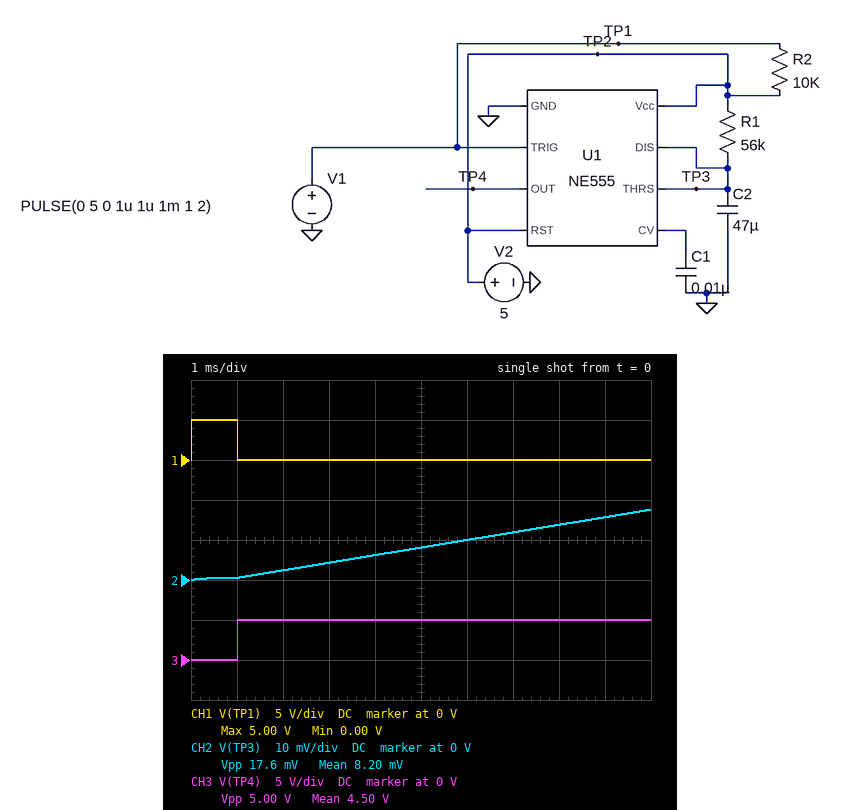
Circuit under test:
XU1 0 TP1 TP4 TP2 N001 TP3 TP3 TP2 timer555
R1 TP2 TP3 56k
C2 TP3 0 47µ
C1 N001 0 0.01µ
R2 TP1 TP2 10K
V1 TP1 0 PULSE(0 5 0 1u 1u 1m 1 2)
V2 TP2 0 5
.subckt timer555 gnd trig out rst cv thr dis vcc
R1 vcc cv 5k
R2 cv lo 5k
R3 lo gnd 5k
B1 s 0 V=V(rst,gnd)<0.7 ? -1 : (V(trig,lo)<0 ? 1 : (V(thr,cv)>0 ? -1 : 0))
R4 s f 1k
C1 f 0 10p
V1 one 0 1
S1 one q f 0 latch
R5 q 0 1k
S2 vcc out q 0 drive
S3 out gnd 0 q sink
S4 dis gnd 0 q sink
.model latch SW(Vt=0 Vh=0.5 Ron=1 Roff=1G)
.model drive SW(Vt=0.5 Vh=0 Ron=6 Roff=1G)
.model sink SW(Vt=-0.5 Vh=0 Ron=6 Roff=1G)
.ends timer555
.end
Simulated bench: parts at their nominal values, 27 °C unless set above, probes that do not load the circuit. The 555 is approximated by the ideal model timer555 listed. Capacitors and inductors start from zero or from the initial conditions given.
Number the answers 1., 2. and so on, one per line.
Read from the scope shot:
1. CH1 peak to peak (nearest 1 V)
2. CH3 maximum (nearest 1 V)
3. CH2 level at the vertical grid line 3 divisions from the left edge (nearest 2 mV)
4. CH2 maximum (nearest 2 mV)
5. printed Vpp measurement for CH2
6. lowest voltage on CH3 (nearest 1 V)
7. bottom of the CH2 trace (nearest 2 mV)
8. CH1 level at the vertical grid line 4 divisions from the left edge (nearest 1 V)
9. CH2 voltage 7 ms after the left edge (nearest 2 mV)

1. 5 V
2. 5 V
3. 4 mV
4. 18 mV
5. 17.6 mV
6. 0 V
7. 0 V
8. 0 V
9. 12 mV
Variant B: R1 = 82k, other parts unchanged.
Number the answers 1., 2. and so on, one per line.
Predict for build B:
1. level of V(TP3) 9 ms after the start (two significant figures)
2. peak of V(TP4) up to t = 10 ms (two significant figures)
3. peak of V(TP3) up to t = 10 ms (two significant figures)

1. 11 mV
2. 5.0 V
3. 12 mV
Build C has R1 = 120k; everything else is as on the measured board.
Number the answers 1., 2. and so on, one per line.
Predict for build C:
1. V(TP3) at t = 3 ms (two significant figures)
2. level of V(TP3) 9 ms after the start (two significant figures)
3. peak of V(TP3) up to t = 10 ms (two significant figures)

1. 2.0 mV
2. 7.3 mV
3. 8.2 mV
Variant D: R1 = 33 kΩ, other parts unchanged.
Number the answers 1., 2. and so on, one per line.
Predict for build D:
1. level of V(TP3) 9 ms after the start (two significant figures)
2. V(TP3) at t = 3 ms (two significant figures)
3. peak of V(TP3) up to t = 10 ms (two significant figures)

1. 27 mV
2. 7.3 mV
3. 30 mV
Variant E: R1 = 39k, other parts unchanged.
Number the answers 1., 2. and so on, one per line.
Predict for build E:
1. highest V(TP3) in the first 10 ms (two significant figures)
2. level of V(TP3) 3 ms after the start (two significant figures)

1. 25 mV
2. 6.2 mV
